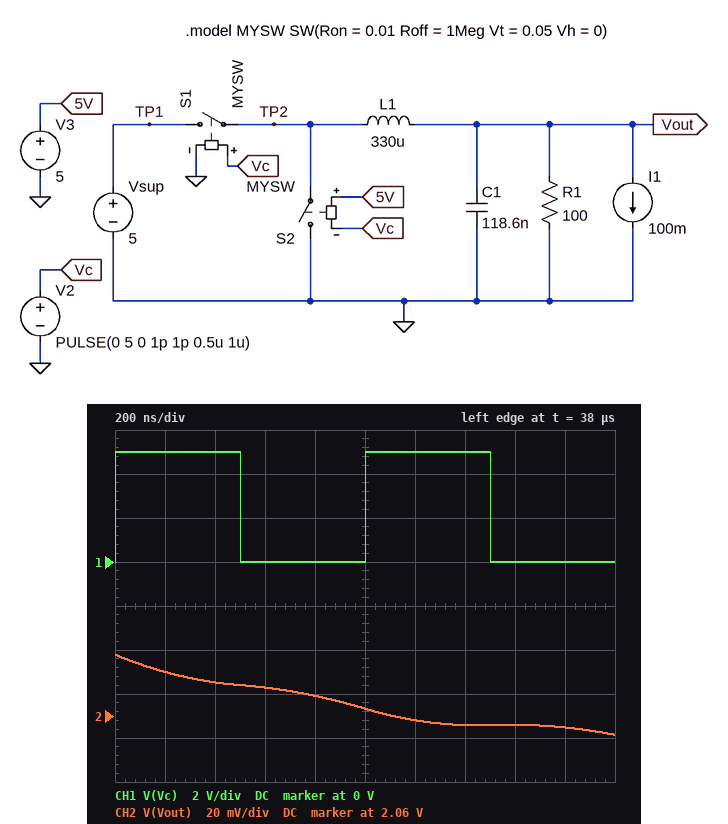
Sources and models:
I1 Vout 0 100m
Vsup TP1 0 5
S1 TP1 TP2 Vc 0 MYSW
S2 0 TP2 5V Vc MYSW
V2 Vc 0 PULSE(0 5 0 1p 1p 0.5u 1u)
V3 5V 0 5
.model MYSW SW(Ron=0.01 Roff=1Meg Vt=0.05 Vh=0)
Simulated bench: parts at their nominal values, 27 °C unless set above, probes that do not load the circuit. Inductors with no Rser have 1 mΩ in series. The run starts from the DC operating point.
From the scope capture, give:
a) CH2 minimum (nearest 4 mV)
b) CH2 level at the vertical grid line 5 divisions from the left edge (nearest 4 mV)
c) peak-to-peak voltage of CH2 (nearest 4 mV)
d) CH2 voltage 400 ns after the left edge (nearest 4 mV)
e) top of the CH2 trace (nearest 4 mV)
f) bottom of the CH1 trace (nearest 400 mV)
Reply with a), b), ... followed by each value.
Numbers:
a) 2.052 V
b) 2.064 V
c) 36 mV
d) 2.076 V
e) 2.088 V
f) 0 V
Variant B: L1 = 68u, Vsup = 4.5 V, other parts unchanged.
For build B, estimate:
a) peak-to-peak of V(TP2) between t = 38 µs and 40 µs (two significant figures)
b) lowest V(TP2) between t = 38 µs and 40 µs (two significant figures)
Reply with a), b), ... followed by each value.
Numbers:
a) 4.5 V
b) -1.5 mV
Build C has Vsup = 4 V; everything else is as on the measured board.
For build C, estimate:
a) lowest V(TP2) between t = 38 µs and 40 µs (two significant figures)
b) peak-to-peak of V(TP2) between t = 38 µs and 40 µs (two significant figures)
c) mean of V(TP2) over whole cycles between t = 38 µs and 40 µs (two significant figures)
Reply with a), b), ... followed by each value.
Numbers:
a) -1.2 mV
b) 4.0 V
c) 2.0 V
